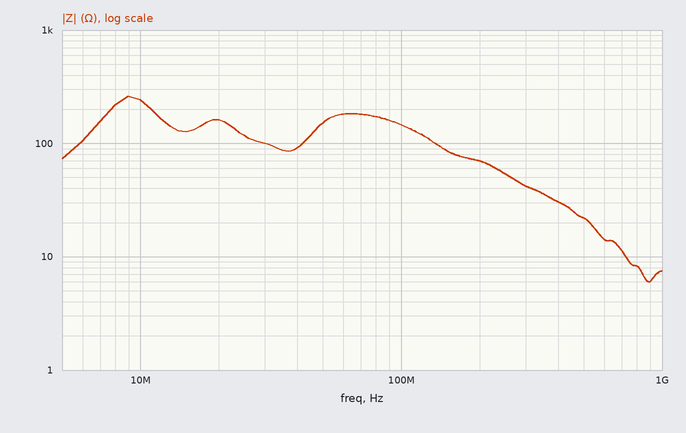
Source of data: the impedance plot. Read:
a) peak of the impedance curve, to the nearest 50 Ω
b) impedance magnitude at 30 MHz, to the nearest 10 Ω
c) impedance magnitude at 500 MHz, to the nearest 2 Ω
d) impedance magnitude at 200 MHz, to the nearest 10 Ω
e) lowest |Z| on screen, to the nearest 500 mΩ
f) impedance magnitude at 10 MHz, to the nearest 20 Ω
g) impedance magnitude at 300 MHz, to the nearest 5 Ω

250 Ω
100 Ω
22 Ω
70 Ω
6.0 Ω
240 Ω
40 Ω
